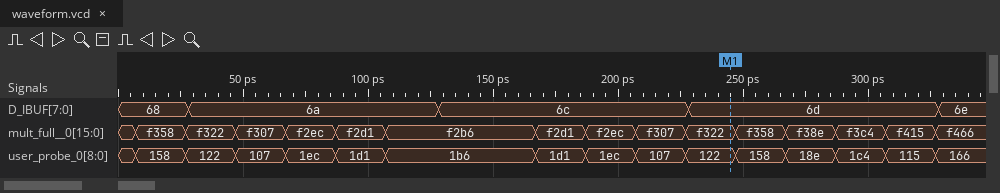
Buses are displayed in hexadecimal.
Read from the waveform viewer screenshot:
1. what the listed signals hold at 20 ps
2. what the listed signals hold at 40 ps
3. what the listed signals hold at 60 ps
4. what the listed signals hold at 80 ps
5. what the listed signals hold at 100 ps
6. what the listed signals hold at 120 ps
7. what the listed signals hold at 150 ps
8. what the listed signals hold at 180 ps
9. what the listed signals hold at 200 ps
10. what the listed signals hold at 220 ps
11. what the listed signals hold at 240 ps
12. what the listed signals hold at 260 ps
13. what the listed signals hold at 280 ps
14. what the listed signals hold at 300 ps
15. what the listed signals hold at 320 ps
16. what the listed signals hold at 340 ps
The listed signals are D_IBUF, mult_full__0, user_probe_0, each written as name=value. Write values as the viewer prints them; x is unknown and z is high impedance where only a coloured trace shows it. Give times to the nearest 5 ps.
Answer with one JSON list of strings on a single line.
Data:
["D_IBUF=68, mult_full__0=f358, user_probe_0=158", "D_IBUF=6a, mult_full__0=f322, user_probe_0=122", "D_IBUF=6a, mult_full__0=f307, user_probe_0=107", "D_IBUF=6a, mult_full__0=f2ec, user_probe_0=1ec", "D_IBUF=6a, mult_full__0=f2d1, user_probe_0=1d1", "D_IBUF=6a, mult_full__0=f2b6, user_probe_0=1b6", "D_IBUF=6c, mult_full__0=f2b6, user_probe_0=1b6", "D_IBUF=6c, mult_full__0=f2d1, user_probe_0=1d1", "D_IBUF=6c, mult_full__0=f2ec, user_probe_0=1ec", "D_IBUF=6c, mult_full__0=f307, user_probe_0=107", "D_IBUF=6d, mult_full__0=f322, user_probe_0=122", "D_IBUF=6d, mult_full__0=f358, user_probe_0=158", "D_IBUF=6d, mult_full__0=f38e, user_probe_0=18e", "D_IBUF=6d, mult_full__0=f3c4, user_probe_0=1c4", "D_IBUF=6d, mult_full__0=f415, user_probe_0=115", "D_IBUF=6e, mult_full__0=f466, user_probe_0=166"]
